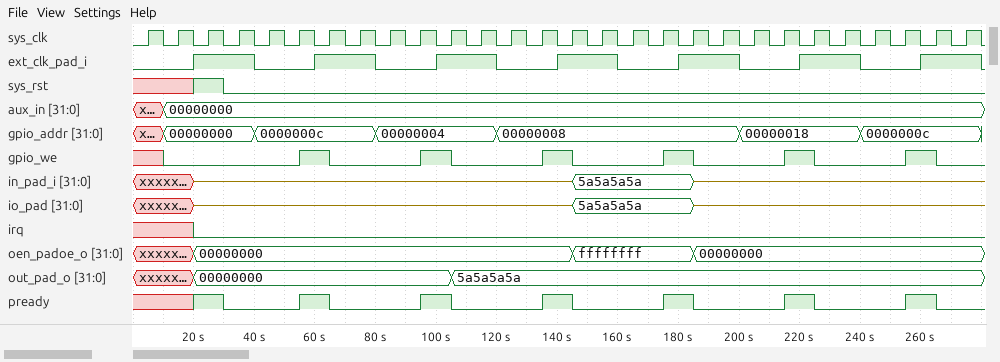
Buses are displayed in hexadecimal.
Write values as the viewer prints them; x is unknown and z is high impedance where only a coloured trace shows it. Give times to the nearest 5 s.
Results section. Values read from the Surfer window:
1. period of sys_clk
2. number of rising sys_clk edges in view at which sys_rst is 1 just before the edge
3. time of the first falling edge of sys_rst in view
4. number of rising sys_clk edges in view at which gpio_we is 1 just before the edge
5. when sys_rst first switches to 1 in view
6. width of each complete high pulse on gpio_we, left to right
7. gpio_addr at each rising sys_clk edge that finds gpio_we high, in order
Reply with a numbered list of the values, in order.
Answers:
1. 10 s
2. 1
3. 30 s
4. 6
5. 20 s
6. 10 s, 10 s, 10 s, 10 s, 10 s, 10 s
7. 0000000c, 00000004, 00000008, 00000008, 00000018, 0000000c
